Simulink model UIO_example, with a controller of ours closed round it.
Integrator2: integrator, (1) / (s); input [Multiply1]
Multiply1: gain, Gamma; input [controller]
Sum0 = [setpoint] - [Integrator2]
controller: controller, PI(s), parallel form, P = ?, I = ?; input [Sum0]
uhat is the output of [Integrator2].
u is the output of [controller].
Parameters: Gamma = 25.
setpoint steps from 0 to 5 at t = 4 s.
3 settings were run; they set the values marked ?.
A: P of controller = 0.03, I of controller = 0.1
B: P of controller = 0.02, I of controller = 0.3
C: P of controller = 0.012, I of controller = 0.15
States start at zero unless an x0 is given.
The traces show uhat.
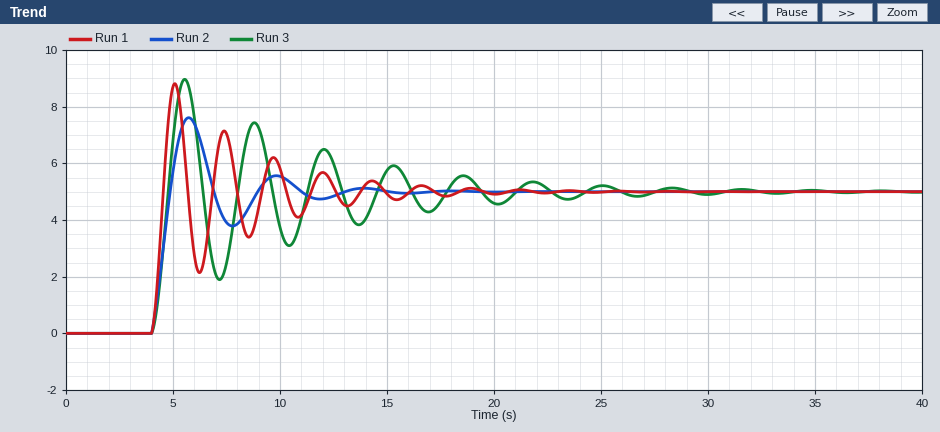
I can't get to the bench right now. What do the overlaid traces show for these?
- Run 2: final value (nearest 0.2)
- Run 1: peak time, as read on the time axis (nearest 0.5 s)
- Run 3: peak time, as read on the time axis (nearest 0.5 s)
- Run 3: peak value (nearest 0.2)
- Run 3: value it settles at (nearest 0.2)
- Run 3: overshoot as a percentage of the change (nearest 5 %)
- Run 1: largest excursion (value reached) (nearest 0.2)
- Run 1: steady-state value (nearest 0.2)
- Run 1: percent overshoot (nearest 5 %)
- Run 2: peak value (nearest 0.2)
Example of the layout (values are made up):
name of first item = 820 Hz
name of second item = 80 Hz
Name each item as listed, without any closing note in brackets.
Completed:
Run 2: final value = 5.0
Run 1: peak time, as read on the time axis = 5.0 s
Run 3: peak time, as read on the time axis = 5.5 s
Run 3: peak value = 9.0
Run 3: value it settles at = 5.0
Run 3: overshoot as a percentage of the change = 80 %
Run 1: largest excursion (value reached) = 8.8
Run 1: steady-state value = 5.0
Run 1: percent overshoot = 75 %
Run 2: peak value = 7.6
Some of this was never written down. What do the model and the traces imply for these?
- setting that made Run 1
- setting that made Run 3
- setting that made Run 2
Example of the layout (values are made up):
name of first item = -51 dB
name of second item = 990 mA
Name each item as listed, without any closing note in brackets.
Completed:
setting that made Run 1 = B
setting that made Run 3 = C
setting that made Run 2 = A
